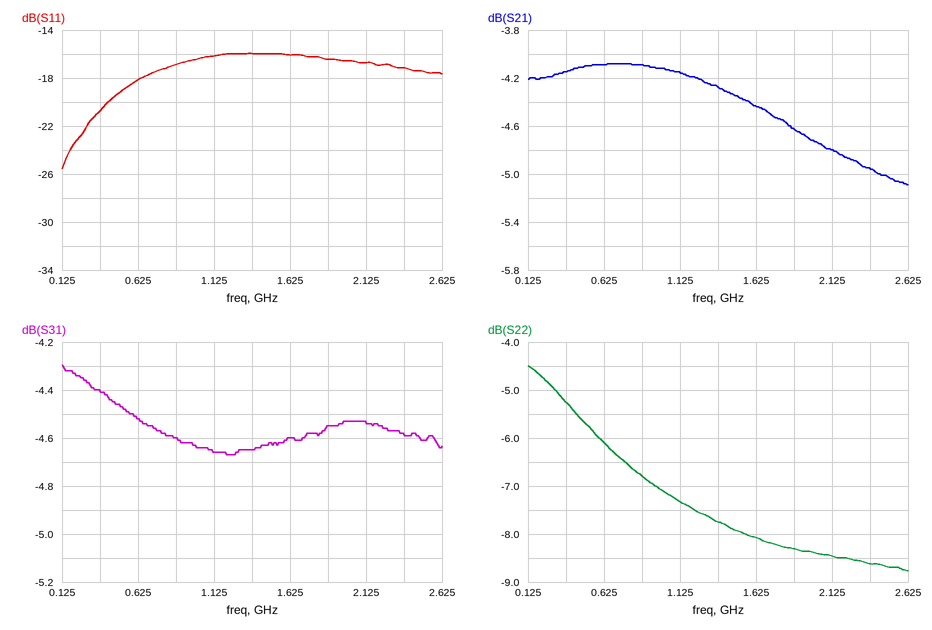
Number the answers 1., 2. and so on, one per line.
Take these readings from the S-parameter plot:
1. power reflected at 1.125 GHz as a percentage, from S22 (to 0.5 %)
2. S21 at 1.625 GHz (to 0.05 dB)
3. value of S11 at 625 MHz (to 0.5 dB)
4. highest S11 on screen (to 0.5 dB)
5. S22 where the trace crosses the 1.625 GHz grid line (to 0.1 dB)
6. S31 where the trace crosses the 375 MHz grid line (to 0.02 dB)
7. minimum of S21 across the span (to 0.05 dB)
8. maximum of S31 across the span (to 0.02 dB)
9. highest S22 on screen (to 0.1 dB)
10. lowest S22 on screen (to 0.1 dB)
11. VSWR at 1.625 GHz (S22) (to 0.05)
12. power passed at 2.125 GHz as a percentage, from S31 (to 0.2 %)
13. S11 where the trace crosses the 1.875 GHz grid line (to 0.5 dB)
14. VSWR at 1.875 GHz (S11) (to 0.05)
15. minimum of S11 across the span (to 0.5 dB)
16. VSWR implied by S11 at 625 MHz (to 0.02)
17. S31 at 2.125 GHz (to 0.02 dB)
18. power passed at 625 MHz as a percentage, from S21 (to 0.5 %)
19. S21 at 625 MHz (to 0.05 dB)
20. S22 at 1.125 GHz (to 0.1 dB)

1. 18.5 %
2. -4.45 dB
3. -18.0 dB
4. -16.0 dB
5. -8.1 dB
6. -4.40 dB
7. -5.10 dB
8. -4.30 dB
9. -4.5 dB
10. -8.8 dB
11. 2.30
12. 35.2 %
13. -16.5 dB
14. 1.35
15. -25.5 dB
16. 1.28
17. -4.54 dB
18. 39.0 %
19. -4.10 dB
20. -7.3 dB
